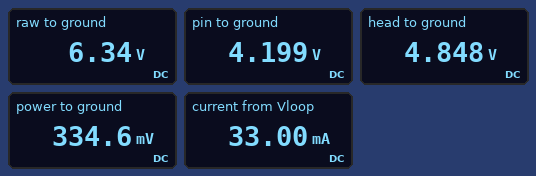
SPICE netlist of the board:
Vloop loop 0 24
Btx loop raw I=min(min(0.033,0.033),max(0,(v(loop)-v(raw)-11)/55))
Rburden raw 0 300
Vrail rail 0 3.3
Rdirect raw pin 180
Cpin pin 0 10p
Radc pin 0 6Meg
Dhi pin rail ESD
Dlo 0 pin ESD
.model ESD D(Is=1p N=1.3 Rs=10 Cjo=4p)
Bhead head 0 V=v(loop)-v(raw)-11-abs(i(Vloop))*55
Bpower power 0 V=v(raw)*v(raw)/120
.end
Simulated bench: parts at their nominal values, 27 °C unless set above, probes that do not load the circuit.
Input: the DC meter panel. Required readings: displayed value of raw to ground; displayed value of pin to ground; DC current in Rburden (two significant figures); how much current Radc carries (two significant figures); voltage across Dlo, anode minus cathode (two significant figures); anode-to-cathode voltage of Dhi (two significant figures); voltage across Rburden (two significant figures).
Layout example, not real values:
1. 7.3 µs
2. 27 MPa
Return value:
1. 6.34 V
2. 4.199 V
3. 21 mA
4. 700 nA
5. -4.2 V
6. 900 mV
7. 6.3 V
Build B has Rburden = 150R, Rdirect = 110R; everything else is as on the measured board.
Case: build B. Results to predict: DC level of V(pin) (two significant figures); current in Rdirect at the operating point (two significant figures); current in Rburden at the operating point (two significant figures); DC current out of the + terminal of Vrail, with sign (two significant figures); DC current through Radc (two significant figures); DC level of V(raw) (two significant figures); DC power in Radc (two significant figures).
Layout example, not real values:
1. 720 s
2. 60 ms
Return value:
1. 4.1 V
2. 3.4 mA
3. 30 mA
4. -3.4 mA
5. 680 nA
6. 4.4 V
7. 2.8 µW
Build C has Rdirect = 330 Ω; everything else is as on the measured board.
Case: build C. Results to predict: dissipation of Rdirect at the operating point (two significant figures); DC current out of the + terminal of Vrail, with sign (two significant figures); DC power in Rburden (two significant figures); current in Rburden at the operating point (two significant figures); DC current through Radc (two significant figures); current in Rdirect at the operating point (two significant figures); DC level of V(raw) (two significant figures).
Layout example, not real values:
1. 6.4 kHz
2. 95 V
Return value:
1. 27 mW
2. -9.1 mA
3. 170 mW
4. 24 mA
5. 690 nA
6. 9.1 mA
7. 7.2 V
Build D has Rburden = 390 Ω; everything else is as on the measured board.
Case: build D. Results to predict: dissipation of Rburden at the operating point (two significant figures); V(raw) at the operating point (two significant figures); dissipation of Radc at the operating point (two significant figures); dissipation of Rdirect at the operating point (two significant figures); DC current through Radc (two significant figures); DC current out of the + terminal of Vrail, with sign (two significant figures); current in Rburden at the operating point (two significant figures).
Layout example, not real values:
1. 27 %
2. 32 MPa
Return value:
1. 120 mW
2. 7.0 V
3. 3.0 µW
4. 41 mW
5. 710 nA
6. -15 mA
7. 18 mA
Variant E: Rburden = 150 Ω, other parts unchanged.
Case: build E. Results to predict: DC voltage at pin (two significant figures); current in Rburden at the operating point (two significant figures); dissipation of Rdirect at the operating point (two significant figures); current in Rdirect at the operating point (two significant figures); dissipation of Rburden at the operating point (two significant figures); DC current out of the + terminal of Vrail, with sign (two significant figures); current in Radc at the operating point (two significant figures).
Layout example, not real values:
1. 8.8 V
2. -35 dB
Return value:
1. 4.1 V
2. 30 mA
3. 1.3 mW
4. 2.7 mA
5. 140 mW
6. -2.7 mA
7. 680 nA
